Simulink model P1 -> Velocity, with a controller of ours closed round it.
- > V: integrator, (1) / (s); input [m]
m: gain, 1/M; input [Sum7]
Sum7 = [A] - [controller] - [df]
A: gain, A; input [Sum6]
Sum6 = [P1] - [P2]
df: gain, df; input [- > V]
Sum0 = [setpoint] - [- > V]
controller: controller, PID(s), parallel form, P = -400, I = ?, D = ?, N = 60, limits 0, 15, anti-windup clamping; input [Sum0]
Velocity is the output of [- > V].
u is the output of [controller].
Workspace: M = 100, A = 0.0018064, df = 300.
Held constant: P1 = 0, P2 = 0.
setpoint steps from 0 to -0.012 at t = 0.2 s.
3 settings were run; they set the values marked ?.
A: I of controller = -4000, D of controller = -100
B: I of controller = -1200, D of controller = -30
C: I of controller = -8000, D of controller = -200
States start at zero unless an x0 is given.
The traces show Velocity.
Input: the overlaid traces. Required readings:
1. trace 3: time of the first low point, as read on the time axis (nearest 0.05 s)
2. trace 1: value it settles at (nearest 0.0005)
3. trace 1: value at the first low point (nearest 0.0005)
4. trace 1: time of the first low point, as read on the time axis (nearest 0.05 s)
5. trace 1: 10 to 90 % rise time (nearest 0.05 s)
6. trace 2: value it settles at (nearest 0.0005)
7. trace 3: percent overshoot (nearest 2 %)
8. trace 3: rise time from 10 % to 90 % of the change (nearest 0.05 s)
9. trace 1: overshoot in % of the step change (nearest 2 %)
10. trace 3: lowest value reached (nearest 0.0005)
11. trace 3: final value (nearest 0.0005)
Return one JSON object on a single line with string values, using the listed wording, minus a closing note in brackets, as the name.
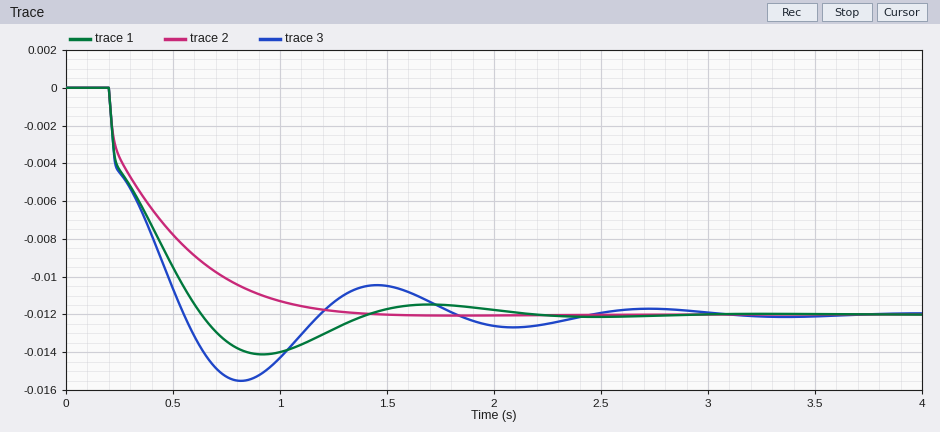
{"trace 3: time of the first low point, as read on the time axis": "0.80 s", "trace 1: value it settles at": "-0.0120", "trace 1: value at the first low point": "-0.0140", "trace 1: time of the first low point, as read on the time axis": "0.90 s", "trace 1: 10 to 90 % rise time": "0.35 s", "trace 2: value it settles at": "-0.0120", "trace 3: percent overshoot": "30 %", "trace 3: rise time from 10 % to 90 % of the change": "0.30 s", "trace 1: overshoot in % of the step change": "18 %", "trace 3: lowest value reached": "-0.0155", "trace 3: final value": "-0.0120"}
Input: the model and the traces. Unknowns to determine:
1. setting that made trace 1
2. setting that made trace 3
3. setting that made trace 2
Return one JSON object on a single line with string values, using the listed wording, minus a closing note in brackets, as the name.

{"setting that made trace 1": "A", "setting that made trace 3": "C", "setting that made trace 2": "B"}
